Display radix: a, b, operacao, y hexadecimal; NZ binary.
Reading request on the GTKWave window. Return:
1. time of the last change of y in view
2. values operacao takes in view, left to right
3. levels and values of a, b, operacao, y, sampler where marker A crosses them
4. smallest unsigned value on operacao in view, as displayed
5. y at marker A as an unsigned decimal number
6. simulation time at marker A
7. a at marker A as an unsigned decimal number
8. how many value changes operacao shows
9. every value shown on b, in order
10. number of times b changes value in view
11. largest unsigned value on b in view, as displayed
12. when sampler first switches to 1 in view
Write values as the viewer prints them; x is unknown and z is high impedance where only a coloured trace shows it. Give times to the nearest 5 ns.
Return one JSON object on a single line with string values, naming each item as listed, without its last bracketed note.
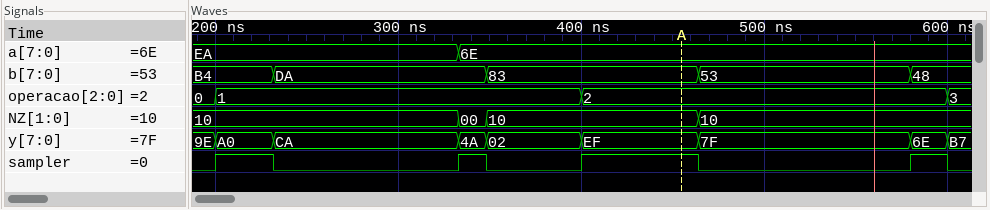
{"time of the last change of y in view": "600 ns", "values operacao takes in view, left to right": "0, 1, 2, 3", "levels and values of a, b, operacao, y, sampler where marker A crosses them": "a=6E, b=83, operacao=2, y=EF, sampler=1", "smallest unsigned value on operacao in view, as displayed": "0", "y at marker A as an unsigned decimal number": "239", "simulation time at marker A": "455 ns", "a at marker A as an unsigned decimal number": "110", "how many value changes operacao shows": "3", "every value shown on b, in order": "B4, DA, 83, 53, 48", "number of times b changes value in view": "4", "largest unsigned value on b in view, as displayed": "DA", "when sampler first switches to 1 in view": "200 ns"}
